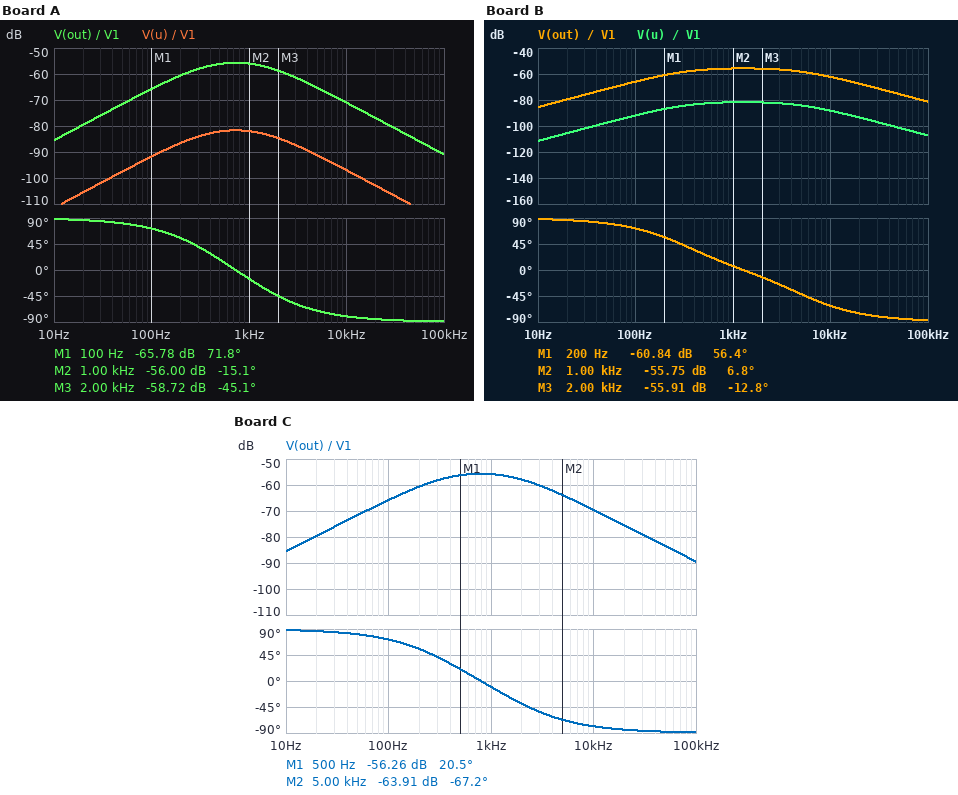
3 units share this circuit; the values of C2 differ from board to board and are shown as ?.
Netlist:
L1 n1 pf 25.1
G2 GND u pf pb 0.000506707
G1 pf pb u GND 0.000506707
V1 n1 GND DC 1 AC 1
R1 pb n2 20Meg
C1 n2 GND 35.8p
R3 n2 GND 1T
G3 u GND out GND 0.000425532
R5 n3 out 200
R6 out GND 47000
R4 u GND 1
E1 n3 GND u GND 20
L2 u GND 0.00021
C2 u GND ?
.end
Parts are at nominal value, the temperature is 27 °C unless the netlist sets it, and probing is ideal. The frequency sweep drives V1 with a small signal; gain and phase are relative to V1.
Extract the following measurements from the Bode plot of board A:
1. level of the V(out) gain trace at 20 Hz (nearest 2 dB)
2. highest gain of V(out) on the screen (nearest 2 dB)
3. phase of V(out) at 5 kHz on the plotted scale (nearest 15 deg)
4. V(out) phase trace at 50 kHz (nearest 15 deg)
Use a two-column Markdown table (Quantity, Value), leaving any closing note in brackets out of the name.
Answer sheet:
| Quantity | Value |
|---|---|
| level of the V(out) gain trace at 20 Hz | -80 dB |
| highest gain of V(out) on the screen | -56 dB |
| phase of V(out) at 5 kHz on the plotted scale | -75 deg |
| V(out) phase trace at 50 kHz | -90 deg |
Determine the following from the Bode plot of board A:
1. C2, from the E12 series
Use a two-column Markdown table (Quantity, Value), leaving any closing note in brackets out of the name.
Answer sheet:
| Quantity | Value |
|---|---|
| C2, from the E12 series | 560 µF |
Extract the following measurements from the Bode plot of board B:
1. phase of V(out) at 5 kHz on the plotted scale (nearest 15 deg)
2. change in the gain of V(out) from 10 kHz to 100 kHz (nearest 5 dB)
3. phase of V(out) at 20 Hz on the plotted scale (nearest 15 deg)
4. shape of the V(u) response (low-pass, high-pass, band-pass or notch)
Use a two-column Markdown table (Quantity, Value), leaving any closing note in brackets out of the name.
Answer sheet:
| Quantity | Value |
|---|---|
| phase of V(out) at 5 kHz on the plotted scale | -45 deg |
| change in the gain of V(out) from 10 kHz to 100 kHz | -20 dB |
| phase of V(out) at 20 Hz on the plotted scale | 90 deg |
| shape of the V(u) response | band-pass |
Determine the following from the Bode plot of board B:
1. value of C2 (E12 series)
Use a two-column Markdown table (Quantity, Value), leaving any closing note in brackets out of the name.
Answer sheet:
| Quantity | Value |
|---|---|
| value of C2 | 180 µF |
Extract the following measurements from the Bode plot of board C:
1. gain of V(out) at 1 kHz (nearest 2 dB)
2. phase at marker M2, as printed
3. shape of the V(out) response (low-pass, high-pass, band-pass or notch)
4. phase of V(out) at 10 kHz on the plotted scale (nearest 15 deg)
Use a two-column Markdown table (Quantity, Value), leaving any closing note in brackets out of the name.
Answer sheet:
| Quantity | Value |
|---|---|
| gain of V(out) at 1 kHz | -56 dB |
| phase at marker M2, as printed | -67.2 deg |
| shape of the V(out) response | band-pass |
| phase of V(out) at 10 kHz on the plotted scale | -75 deg |
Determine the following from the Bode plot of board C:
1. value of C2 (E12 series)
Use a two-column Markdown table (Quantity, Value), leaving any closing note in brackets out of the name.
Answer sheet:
| Quantity | Value |
|---|---|
| value of C2 | 470 µF |
